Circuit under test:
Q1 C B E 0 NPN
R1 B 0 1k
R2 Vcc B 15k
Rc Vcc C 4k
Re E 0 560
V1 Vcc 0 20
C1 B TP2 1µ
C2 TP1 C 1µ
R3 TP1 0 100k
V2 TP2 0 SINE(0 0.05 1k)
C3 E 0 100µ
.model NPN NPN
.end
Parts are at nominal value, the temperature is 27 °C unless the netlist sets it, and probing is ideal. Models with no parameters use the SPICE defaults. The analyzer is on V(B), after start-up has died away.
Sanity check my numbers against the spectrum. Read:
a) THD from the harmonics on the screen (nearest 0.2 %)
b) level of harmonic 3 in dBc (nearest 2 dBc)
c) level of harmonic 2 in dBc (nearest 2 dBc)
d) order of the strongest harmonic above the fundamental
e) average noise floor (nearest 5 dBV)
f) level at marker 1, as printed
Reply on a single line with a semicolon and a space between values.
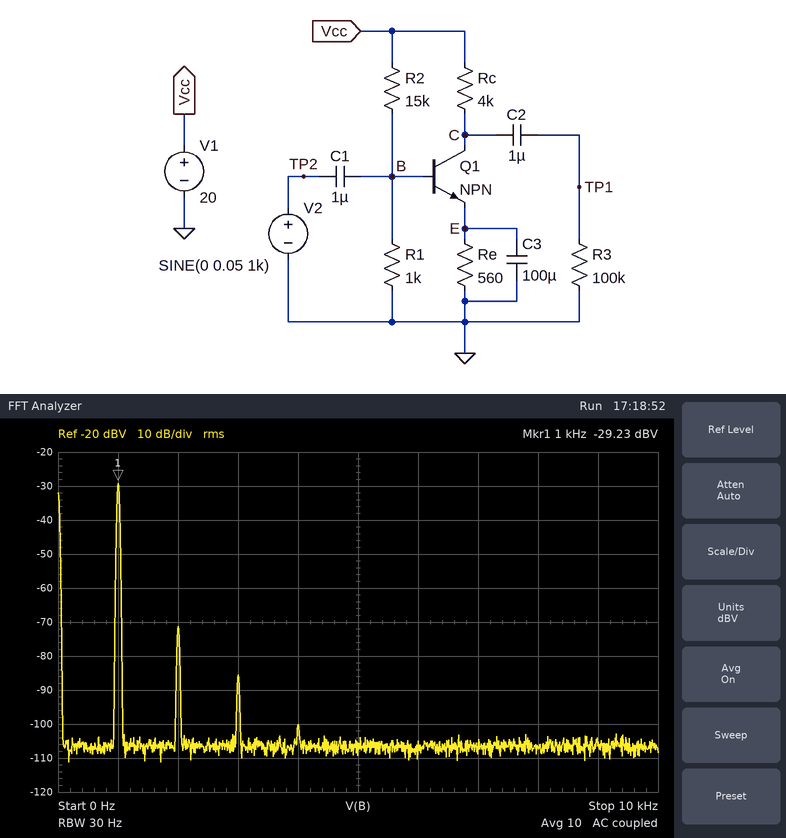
0.8 %; -56 dBc; -42 dBc; 2; -105 dBV; -29.23 dBV
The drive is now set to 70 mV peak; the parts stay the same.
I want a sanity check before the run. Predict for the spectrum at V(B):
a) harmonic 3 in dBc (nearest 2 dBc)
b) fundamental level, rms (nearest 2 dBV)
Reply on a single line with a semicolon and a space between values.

-54 dBc; -26 dBV
